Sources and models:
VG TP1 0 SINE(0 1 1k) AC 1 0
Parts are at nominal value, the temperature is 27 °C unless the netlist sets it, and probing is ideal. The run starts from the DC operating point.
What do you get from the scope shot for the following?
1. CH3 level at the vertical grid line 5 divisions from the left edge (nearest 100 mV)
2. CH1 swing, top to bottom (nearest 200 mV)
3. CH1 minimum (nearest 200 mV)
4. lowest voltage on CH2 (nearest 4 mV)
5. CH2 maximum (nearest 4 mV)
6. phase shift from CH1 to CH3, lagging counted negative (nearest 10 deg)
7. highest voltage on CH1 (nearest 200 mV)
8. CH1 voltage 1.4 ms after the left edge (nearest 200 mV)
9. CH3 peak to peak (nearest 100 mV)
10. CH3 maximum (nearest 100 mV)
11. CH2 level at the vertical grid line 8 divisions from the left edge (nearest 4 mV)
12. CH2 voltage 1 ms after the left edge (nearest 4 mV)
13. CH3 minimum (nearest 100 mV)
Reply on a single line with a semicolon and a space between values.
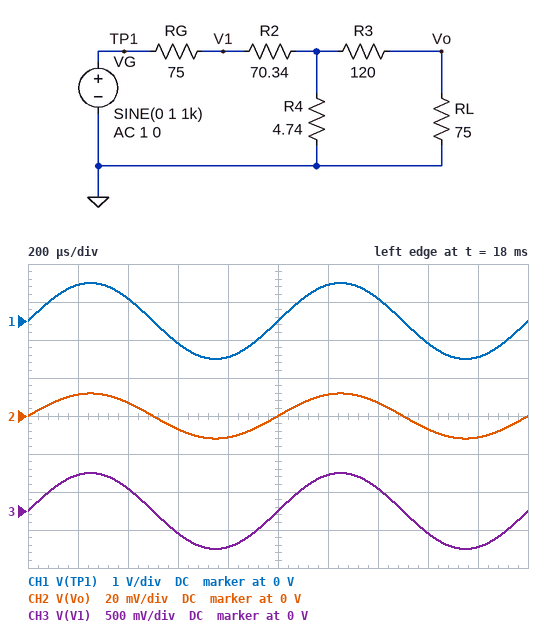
0 V; 2.0 V; -1.0 V; -12 mV; 12 mV; 0 deg; 1.0 V; 600 mV; 1.0 V; 500 mV; -8 mV; 0 V; -500 mV
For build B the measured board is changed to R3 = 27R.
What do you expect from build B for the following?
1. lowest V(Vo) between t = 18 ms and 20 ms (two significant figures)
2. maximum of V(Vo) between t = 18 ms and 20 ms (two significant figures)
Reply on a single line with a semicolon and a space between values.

-22 mV; 22 mV
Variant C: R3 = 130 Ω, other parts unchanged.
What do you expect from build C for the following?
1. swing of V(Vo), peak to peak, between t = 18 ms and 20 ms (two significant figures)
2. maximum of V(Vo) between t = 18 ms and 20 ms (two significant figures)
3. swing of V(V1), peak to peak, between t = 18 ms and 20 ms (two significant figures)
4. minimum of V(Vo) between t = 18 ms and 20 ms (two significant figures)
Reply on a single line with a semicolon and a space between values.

23 mV; 11 mV; 1.0 V; -11 mV
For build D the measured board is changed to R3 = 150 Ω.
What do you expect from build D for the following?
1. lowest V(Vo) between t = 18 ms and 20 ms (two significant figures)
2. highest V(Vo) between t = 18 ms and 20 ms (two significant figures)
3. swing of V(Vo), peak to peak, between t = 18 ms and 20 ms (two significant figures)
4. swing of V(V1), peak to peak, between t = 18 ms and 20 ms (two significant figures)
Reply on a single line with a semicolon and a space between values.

-10 mV; 10 mV; 21 mV; 1.0 V
